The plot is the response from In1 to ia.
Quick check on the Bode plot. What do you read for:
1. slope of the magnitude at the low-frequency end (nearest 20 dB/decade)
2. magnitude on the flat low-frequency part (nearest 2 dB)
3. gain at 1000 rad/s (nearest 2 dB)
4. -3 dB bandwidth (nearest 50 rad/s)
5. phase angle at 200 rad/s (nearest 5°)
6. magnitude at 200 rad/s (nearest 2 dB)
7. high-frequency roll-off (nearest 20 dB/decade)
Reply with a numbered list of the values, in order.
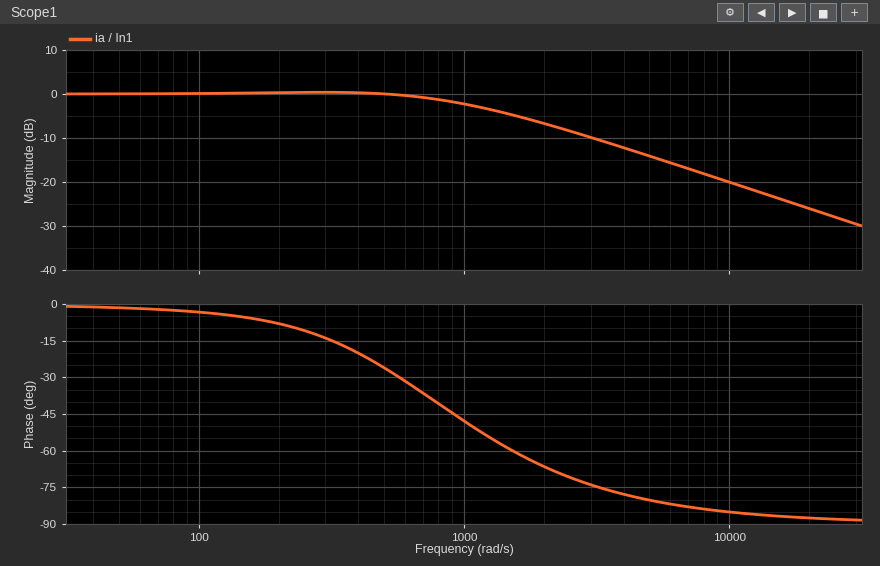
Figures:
1. 0 dB/decade
2. 0 dB
3. -2 dB
4. 1150 rad/s
5. -10°
6. 0 dB
7. -20 dB/decade
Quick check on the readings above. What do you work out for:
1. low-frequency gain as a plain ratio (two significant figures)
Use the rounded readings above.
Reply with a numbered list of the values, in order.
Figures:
1. 1.0
